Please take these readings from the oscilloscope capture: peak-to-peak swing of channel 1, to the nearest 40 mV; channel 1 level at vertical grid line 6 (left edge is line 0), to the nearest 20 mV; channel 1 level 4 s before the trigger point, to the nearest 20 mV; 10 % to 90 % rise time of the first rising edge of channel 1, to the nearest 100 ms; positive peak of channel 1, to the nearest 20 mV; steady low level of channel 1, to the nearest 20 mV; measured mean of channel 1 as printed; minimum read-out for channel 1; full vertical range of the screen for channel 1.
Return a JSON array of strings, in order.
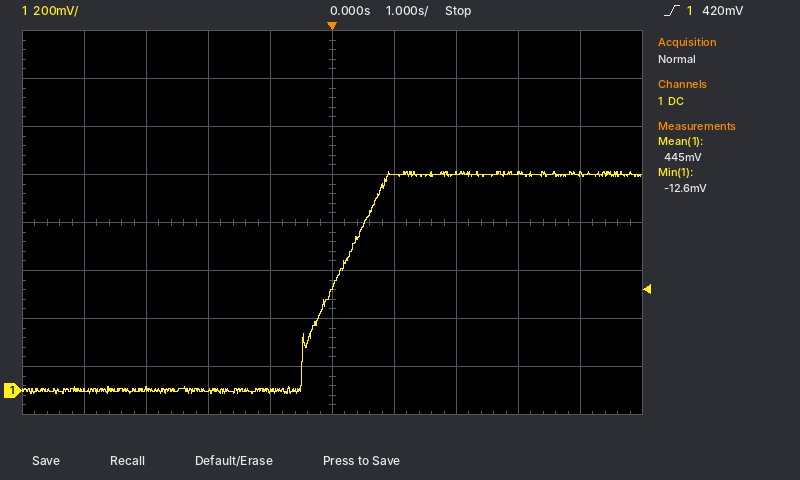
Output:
["920 mV", "900 mV", "0 mV", "1.2 s", "920 mV", "0 mV", "445 mV", "-12.6 mV", "1.6 V"]
